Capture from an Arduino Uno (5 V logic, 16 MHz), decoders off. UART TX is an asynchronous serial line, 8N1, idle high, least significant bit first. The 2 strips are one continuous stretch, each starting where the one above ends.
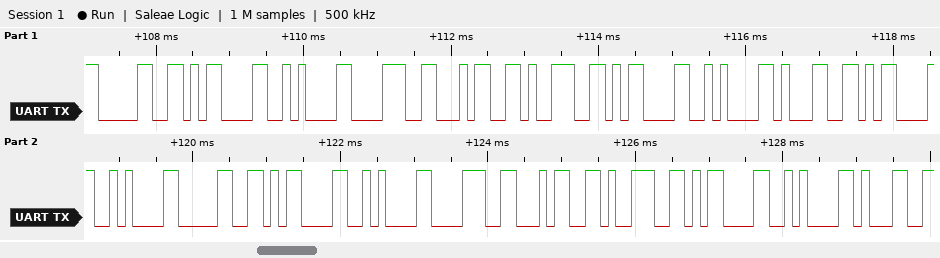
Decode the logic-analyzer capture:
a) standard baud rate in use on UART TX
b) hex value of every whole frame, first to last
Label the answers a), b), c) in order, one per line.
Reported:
a) 9600 baud
b) 0x30 0x0D 0x0A 0x38 0x34 0x39 0x0D 0x0A 0x31 0x0D 0x0A 0x30 0x0D 0x0A 0x38 0x34 0x39 0x0D 0x0A 0x31
